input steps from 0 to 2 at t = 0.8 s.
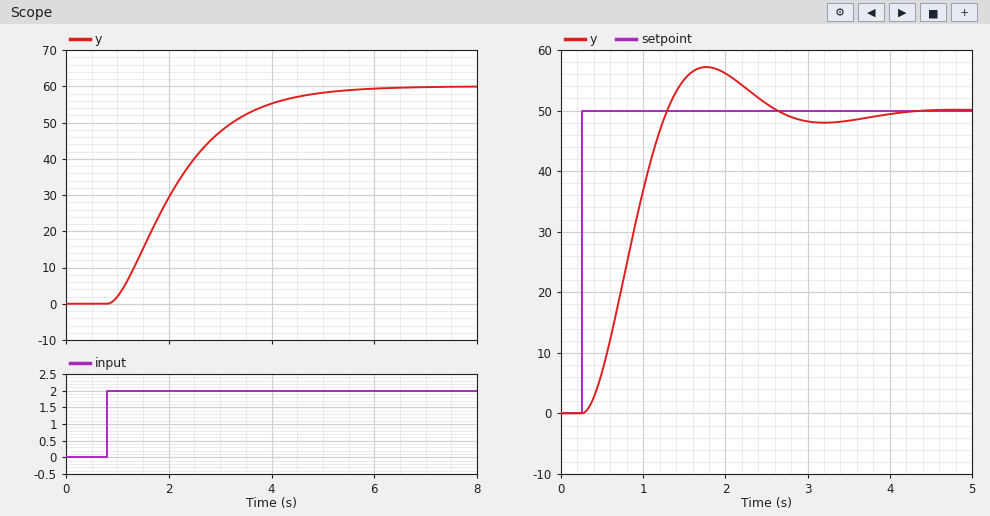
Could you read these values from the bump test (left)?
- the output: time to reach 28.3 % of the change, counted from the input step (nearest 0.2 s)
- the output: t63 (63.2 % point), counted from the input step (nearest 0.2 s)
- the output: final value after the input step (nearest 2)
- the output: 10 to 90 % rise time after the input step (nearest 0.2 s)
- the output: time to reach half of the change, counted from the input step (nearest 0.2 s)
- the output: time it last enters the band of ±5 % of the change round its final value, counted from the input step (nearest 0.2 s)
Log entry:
0.8 s
1.6 s
60
2.6 s
1.2 s
3.6 s
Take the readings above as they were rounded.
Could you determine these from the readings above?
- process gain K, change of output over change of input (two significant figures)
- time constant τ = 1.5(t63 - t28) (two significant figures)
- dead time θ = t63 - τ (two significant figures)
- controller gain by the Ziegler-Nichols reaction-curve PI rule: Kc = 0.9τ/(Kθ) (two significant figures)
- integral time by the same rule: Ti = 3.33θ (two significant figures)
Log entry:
30
1.2 s
0.40 s
0.090
1.3 s
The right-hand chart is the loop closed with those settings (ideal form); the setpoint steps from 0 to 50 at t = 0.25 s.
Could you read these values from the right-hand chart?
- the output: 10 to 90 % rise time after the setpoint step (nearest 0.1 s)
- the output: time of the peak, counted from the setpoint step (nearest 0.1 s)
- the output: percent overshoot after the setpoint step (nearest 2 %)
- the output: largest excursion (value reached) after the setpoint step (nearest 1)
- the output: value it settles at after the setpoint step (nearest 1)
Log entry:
0.7 s
1.5 s
14 %
57
50
